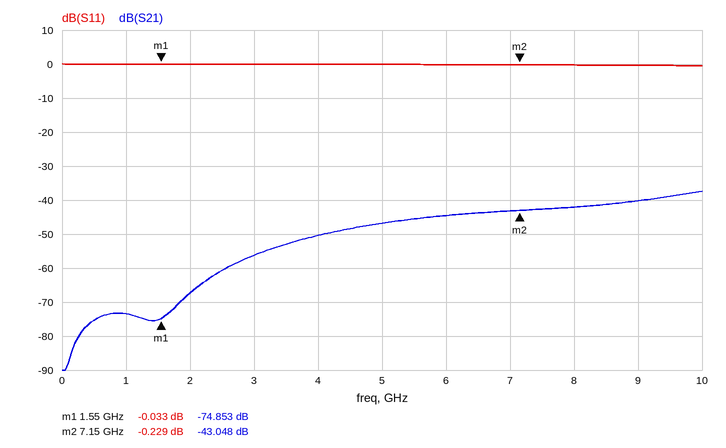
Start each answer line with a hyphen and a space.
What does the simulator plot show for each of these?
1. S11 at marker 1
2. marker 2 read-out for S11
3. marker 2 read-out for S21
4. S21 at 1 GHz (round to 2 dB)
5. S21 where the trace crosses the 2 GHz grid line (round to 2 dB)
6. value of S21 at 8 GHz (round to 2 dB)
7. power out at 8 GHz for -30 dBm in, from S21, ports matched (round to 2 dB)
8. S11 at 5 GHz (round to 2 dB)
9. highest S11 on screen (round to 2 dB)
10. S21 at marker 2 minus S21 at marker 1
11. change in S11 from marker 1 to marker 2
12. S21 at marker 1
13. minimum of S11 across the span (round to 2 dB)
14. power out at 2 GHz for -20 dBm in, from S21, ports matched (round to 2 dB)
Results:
- -0.033 dB
- -0.229 dB
- -43.048 dB
- -74 dB
- -68 dB
- -42 dB
- -72 dBm
- 0 dB
- 0 dB
- 31.805 dB
- -0.196 dB
- -74.853 dB
- 0 dB
- -88 dBm
